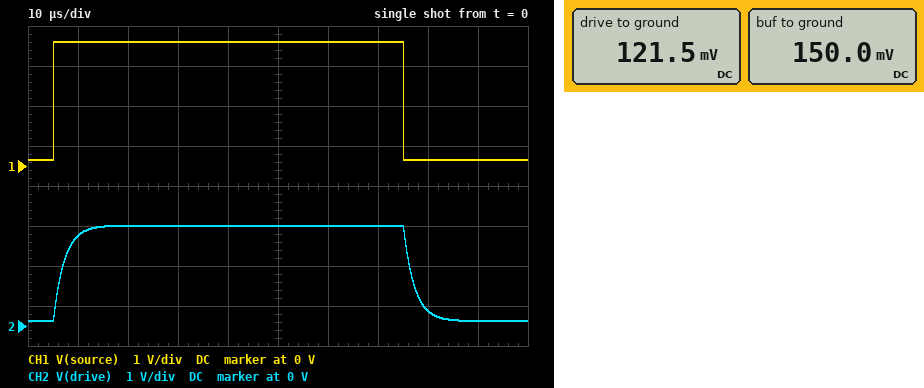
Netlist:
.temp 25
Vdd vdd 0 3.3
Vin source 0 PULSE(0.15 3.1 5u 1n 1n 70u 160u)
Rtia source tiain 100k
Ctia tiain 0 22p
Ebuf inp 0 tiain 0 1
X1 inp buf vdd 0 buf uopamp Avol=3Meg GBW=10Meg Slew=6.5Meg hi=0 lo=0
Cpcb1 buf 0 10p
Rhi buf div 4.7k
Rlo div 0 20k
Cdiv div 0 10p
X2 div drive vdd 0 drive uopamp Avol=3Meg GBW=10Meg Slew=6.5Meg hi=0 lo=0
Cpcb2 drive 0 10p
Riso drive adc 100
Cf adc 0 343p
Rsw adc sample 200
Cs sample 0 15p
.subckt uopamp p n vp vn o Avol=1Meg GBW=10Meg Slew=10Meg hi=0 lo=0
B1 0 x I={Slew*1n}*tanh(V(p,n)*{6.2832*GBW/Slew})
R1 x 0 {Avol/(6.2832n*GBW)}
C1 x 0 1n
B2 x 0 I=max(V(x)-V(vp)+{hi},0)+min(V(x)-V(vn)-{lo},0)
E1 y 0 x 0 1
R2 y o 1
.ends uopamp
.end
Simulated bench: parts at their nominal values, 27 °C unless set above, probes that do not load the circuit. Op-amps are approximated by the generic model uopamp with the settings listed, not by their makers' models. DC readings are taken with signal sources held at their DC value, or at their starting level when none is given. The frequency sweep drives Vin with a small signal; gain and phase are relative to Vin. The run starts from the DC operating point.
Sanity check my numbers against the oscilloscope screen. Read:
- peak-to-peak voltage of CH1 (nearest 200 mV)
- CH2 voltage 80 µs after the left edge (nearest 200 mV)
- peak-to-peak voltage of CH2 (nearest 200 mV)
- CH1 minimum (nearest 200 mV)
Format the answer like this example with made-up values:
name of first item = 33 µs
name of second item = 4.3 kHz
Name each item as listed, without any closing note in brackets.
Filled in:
peak-to-peak voltage of CH1 = 3.0 V
CH2 voltage 80 µs after the left edge = 400 mV
peak-to-peak voltage of CH2 = 2.4 V
CH1 minimum = 200 mV
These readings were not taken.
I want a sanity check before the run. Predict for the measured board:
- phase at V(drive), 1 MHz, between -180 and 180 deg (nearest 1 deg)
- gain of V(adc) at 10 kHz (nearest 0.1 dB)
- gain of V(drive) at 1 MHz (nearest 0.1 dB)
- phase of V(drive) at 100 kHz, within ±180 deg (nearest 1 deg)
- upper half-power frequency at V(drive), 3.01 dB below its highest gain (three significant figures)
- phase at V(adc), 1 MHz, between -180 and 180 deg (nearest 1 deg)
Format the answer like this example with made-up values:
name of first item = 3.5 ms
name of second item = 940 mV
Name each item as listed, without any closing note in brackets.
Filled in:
phase at V(drive), 1 MHz, between -180 and 180 deg = -111 deg
gain of V(adc) at 10 kHz = -1.9 dB
gain of V(drive) at 1 MHz = -25.0 dB
phase of V(drive) at 100 kHz, within ±180 deg = -57 deg
upper half-power frequency at V(drive), 3.01 dB below its highest gain = 72.3 kHz
phase at V(adc), 1 MHz, between -180 and 180 deg = -123 deg
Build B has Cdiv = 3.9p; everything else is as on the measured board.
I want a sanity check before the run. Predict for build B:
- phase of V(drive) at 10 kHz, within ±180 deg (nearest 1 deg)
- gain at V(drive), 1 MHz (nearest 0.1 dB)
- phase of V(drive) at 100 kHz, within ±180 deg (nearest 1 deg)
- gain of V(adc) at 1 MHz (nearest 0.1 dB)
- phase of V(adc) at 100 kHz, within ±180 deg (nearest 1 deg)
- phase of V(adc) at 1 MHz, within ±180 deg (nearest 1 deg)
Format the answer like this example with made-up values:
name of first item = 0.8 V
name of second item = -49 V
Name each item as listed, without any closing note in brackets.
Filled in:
phase of V(drive) at 10 kHz, within ±180 deg = -8 deg
gain at V(drive), 1 MHz = -24.8 dB
phase of V(drive) at 100 kHz, within ±180 deg = -56 deg
gain of V(adc) at 1 MHz = -25.0 dB
phase of V(adc) at 100 kHz, within ±180 deg = -57 deg
phase of V(adc) at 1 MHz, within ±180 deg = -115 deg
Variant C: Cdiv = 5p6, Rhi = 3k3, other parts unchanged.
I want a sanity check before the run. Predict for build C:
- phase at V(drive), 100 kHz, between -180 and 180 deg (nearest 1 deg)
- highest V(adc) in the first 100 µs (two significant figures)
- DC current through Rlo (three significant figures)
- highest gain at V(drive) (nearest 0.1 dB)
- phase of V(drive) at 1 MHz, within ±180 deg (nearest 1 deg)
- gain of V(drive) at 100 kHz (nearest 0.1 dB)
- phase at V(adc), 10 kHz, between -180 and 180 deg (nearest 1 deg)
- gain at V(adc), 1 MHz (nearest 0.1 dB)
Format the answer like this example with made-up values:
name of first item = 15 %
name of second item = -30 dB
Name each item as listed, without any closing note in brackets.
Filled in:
phase at V(drive), 100 kHz, between -180 and 180 deg = -56 deg
highest V(adc) in the first 100 µs = 2.7 V
DC current through Rlo = 6.44 µA
highest gain at V(drive) = -1.3 dB
phase of V(drive) at 1 MHz, within ±180 deg = -103 deg
gain of V(drive) at 100 kHz = -6.0 dB
phase at V(adc), 10 kHz, between -180 and 180 deg = -8 deg
gain at V(adc), 1 MHz = -24.5 dB
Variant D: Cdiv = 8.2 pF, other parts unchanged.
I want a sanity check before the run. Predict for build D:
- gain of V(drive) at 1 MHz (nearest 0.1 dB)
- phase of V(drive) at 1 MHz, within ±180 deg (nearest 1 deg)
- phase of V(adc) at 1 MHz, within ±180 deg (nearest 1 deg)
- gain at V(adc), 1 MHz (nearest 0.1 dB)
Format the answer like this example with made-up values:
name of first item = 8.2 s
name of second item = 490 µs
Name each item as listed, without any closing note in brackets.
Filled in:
gain of V(drive) at 1 MHz = -24.9 dB
phase of V(drive) at 1 MHz, within ±180 deg = -108 deg
phase of V(adc) at 1 MHz, within ±180 deg = -121 deg
gain at V(adc), 1 MHz = -25.1 dB
